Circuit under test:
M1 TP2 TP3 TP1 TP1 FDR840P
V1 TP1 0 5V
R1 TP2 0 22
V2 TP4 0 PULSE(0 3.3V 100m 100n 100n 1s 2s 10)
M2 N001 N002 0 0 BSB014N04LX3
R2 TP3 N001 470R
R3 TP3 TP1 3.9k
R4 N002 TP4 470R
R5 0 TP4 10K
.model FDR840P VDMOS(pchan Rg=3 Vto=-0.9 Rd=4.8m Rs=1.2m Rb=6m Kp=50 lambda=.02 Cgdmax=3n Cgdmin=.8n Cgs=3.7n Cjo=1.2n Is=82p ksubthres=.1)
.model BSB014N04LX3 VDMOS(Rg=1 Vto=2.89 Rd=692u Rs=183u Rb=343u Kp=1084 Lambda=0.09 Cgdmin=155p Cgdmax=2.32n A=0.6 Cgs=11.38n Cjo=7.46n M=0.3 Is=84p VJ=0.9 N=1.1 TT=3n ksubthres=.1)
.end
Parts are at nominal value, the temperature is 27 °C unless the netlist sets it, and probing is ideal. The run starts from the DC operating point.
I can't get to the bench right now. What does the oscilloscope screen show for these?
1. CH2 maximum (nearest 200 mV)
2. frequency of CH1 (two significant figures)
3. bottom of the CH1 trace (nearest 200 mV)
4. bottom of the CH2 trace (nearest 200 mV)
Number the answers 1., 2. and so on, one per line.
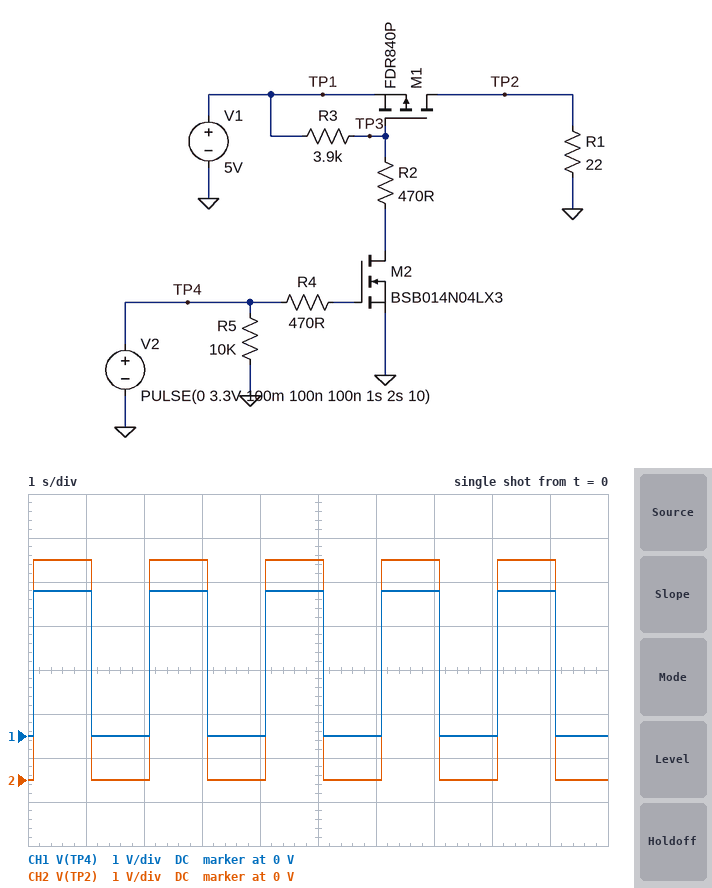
1. 5.0 V
2. 500 mHz
3. 0 V
4. 0 V
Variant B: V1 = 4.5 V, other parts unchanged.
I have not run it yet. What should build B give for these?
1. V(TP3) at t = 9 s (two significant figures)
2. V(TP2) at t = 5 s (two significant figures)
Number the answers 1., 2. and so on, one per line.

1. 480 mV
2. 4.5 V
